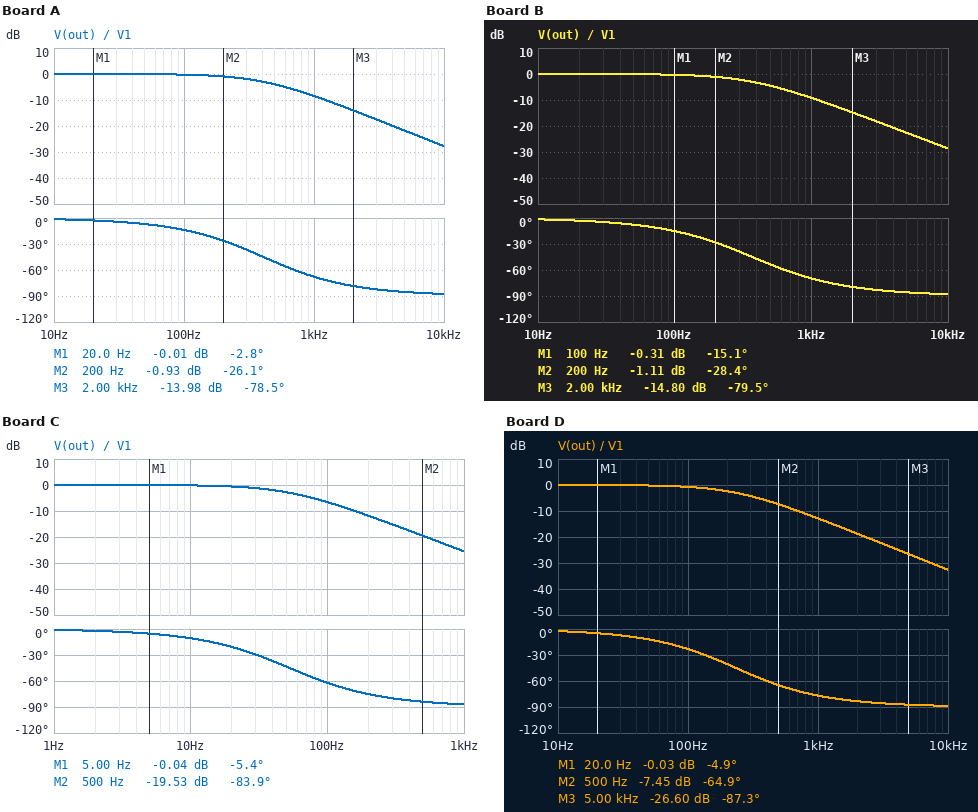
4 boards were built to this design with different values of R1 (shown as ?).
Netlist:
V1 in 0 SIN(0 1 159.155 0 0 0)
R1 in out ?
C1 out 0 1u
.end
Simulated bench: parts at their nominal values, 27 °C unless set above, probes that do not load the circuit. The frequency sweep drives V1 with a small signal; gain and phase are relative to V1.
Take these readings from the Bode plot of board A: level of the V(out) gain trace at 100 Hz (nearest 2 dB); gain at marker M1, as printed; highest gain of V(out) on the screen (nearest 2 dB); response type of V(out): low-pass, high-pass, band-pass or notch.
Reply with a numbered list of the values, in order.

1. 0 dB
2. -0.01 dB
3. 0 dB
4. low-pass
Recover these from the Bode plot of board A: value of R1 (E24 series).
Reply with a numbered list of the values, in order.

1. 390 Ω
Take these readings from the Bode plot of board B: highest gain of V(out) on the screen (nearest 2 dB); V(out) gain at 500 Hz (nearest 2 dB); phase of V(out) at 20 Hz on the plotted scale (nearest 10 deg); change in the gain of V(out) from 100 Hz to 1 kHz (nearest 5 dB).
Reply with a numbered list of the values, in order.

1. 0 dB
2. -4 dB
3. 0 deg
4. -10 dB
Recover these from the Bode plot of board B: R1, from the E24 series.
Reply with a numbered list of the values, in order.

1. 430 Ω
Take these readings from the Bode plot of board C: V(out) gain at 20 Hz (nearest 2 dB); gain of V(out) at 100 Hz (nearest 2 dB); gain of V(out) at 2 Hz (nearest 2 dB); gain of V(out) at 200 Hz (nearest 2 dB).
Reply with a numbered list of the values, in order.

1. 0 dB
2. -6 dB
3. 0 dB
4. -12 dB
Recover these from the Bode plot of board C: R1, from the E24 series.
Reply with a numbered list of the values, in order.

1. 3 kΩ
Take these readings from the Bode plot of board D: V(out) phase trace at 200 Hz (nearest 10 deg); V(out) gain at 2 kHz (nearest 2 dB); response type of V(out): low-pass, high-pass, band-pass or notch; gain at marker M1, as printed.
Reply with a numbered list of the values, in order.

1. -40 deg
2. -18 dB
3. low-pass
4. -0.03 dB
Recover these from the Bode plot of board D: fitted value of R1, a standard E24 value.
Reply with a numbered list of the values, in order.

1. 680 Ω
